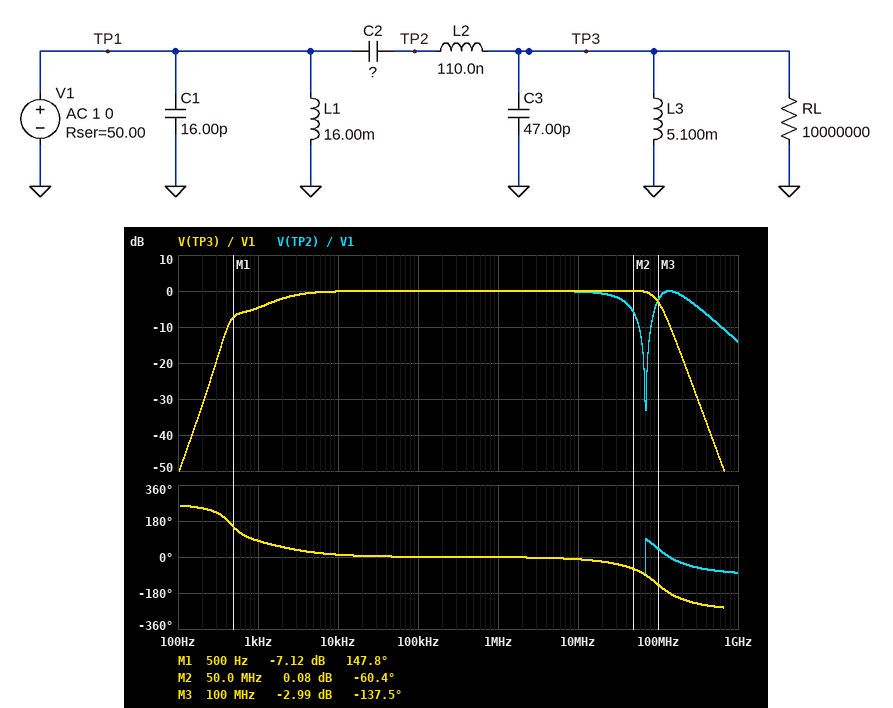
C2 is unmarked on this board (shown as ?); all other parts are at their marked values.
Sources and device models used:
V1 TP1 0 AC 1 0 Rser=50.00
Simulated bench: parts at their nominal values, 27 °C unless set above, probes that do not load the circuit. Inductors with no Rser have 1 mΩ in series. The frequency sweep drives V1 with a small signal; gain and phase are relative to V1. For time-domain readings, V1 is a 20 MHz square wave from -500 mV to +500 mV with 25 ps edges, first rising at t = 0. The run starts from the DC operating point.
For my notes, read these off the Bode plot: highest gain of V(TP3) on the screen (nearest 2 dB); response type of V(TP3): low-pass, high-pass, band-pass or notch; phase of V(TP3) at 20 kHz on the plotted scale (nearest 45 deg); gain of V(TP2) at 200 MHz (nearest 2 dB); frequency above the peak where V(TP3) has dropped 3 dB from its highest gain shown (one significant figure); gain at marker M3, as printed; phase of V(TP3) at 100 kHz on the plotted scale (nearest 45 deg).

0 dB
band-pass
0 deg
-2 dB
100 MHz
-2.99 dB
0 deg
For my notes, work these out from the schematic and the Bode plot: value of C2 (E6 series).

6.8 µF
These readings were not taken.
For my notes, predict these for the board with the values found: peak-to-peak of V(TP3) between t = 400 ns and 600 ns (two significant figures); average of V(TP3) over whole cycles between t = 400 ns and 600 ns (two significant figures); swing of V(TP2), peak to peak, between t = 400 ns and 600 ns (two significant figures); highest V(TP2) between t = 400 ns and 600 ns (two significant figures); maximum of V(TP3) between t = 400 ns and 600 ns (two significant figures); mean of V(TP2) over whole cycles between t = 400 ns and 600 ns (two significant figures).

1.2 V
500 mV
1.1 V
1.1 V
1.1 V
500 mV
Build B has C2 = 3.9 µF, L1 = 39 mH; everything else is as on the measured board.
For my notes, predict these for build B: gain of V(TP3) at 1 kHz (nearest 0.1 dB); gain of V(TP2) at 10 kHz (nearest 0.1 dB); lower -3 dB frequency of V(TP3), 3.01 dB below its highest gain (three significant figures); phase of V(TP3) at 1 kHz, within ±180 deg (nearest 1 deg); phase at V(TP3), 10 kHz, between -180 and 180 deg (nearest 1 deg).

-3.7 dB
0 dB
1.11 kHz
100 deg
10 deg
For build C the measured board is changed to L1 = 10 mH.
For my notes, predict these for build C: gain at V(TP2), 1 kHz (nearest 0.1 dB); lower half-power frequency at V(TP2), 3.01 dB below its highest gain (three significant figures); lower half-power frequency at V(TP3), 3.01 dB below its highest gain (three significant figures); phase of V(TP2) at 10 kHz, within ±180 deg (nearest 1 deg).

-5.1 dB
1.87 kHz
1.91 kHz
13 deg
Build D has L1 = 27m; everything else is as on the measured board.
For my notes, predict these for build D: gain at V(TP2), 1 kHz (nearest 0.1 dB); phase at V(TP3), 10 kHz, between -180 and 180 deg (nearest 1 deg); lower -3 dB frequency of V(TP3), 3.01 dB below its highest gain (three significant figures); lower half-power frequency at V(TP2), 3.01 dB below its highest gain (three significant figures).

-4.4 dB
11 deg
1.39 kHz
1.36 kHz
